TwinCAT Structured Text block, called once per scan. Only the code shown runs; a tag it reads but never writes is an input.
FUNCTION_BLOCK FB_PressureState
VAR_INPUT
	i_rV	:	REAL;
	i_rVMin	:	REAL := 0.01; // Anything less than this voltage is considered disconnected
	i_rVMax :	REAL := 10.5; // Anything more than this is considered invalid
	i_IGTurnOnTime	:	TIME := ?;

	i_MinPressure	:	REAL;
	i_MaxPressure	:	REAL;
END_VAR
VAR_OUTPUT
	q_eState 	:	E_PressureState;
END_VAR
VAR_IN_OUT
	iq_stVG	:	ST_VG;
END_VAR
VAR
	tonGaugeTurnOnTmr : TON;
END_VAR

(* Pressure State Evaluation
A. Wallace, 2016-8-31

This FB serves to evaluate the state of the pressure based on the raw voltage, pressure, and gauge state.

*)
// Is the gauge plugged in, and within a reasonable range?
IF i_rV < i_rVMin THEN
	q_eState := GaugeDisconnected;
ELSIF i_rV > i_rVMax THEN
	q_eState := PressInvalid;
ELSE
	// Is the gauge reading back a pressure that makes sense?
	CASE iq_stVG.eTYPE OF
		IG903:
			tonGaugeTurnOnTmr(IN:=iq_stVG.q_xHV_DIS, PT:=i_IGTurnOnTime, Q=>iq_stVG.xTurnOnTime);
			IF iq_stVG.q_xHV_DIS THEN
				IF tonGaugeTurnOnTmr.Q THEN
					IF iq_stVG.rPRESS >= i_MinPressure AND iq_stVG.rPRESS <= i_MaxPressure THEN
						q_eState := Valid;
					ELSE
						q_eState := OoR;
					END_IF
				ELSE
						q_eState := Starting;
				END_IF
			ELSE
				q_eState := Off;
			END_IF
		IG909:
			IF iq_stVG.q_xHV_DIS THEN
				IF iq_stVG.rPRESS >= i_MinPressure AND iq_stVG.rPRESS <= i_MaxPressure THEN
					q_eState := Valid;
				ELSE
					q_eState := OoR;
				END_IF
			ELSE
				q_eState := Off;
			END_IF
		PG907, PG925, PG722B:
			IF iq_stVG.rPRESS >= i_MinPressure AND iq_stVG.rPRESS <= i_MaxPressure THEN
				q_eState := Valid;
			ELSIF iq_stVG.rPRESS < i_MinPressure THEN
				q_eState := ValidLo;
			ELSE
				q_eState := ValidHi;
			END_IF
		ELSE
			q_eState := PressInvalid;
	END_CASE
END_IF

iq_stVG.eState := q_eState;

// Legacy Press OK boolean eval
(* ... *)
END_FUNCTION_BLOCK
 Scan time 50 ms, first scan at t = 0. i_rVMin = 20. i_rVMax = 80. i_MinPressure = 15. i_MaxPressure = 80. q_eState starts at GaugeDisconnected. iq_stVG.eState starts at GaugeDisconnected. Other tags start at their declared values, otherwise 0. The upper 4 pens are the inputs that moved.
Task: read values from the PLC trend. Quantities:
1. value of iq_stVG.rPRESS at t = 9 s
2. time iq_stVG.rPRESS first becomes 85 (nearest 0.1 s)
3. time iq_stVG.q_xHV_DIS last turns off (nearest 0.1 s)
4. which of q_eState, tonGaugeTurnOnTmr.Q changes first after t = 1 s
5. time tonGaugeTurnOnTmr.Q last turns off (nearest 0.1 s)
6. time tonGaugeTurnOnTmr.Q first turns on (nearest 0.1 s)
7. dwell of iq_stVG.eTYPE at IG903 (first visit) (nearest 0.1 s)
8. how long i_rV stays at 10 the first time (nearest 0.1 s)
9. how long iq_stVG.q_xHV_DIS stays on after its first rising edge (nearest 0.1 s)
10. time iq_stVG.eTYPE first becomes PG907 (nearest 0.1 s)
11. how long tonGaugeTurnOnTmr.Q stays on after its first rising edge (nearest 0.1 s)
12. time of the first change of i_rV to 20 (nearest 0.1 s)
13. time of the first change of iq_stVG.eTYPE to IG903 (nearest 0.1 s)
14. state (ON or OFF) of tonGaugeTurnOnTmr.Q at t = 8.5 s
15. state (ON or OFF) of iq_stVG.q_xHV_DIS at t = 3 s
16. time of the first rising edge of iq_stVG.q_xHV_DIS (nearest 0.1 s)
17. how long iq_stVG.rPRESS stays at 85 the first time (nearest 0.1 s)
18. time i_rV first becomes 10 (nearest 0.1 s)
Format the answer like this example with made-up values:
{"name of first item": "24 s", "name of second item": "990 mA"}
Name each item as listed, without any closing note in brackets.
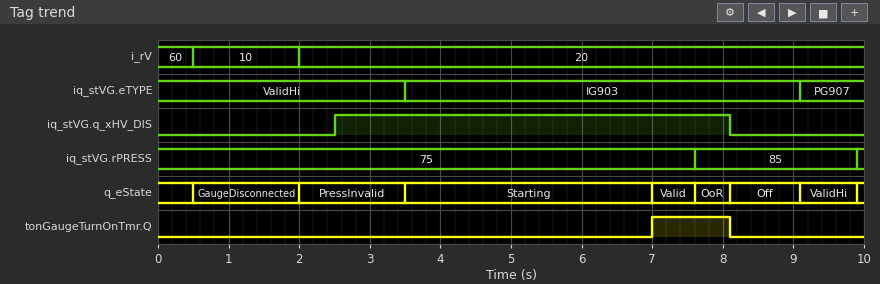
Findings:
{"value of iq_stVG.rPRESS at t = 9 s": "85", "time iq_stVG.rPRESS first becomes 85": "7.6 s", "time iq_stVG.q_xHV_DIS last turns off": "8.1 s", "which of q_eState, tonGaugeTurnOnTmr.Q changes first after t = 1 s": "q_eState", "time tonGaugeTurnOnTmr.Q last turns off": "8.1 s", "time tonGaugeTurnOnTmr.Q first turns on": "7.0 s", "dwell of iq_stVG.eTYPE at IG903 (first visit)": "5.6 s", "how long i_rV stays at 10 the first time": "1.5 s", "how long iq_stVG.q_xHV_DIS stays on after its first rising edge": "5.6 s", "time iq_stVG.eTYPE first becomes PG907": "9.1 s", "how long tonGaugeTurnOnTmr.Q stays on after its first rising edge": "1.1 s", "time of the first change of i_rV to 20": "2.0 s", "time of the first change of iq_stVG.eTYPE to IG903": "3.5 s", "state (ON or OFF) of tonGaugeTurnOnTmr.Q at t = 8.5 s": "OFF", "state (ON or OFF) of iq_stVG.q_xHV_DIS at t = 3 s": "ON", "time of the first rising edge of iq_stVG.q_xHV_DIS": "2.5 s", "how long iq_stVG.rPRESS stays at 85 the first time": "2.3 s", "time i_rV first becomes 10": "0.5 s"}
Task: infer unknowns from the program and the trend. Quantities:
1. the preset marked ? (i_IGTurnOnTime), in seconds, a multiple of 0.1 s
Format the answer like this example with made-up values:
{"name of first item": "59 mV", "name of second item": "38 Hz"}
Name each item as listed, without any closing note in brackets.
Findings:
{"the preset marked ? (i_IGTurnOnTime), in seconds, a multiple of 0.1 s": "3.5 s"}
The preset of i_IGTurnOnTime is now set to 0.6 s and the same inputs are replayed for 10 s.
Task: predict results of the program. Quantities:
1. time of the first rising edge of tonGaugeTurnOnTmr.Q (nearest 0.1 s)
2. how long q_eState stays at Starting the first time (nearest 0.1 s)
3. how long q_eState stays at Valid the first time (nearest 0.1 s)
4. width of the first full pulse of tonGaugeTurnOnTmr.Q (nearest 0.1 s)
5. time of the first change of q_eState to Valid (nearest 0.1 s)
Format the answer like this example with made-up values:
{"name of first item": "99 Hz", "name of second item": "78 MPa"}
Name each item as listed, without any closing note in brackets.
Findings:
{"time of the first rising edge of tonGaugeTurnOnTmr.Q": "4.1 s", "how long q_eState stays at Starting the first time": "0.6 s", "how long q_eState stays at Valid the first time": "3.5 s", "width of the first full pulse of tonGaugeTurnOnTmr.Q": "4.0 s", "time of the first change of q_eState to Valid": "4.1 s"}
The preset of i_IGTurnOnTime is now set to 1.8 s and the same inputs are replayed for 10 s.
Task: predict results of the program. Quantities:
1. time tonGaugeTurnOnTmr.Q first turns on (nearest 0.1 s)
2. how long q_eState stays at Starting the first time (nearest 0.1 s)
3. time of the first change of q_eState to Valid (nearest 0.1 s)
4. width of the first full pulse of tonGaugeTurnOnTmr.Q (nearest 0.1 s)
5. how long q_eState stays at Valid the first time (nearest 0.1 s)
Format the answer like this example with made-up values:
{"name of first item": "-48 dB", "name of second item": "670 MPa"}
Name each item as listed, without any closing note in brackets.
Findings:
{"time tonGaugeTurnOnTmr.Q first turns on": "5.3 s", "how long q_eState stays at Starting the first time": "1.8 s", "time of the first change of q_eState to Valid": "5.3 s", "width of the first full pulse of tonGaugeTurnOnTmr.Q": "2.8 s", "how long q_eState stays at Valid the first time": "2.3 s"}
